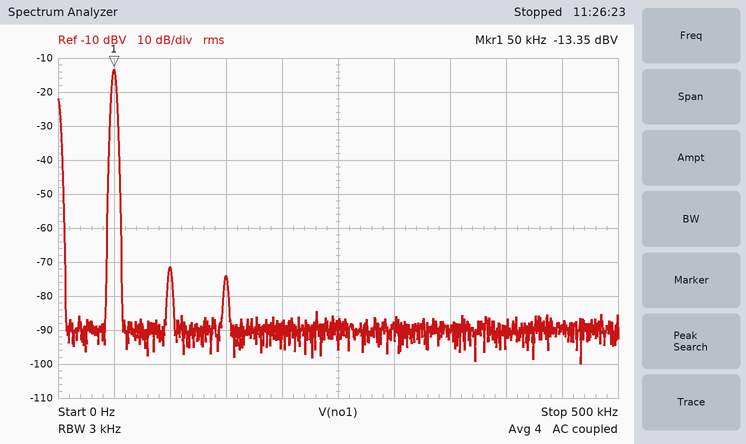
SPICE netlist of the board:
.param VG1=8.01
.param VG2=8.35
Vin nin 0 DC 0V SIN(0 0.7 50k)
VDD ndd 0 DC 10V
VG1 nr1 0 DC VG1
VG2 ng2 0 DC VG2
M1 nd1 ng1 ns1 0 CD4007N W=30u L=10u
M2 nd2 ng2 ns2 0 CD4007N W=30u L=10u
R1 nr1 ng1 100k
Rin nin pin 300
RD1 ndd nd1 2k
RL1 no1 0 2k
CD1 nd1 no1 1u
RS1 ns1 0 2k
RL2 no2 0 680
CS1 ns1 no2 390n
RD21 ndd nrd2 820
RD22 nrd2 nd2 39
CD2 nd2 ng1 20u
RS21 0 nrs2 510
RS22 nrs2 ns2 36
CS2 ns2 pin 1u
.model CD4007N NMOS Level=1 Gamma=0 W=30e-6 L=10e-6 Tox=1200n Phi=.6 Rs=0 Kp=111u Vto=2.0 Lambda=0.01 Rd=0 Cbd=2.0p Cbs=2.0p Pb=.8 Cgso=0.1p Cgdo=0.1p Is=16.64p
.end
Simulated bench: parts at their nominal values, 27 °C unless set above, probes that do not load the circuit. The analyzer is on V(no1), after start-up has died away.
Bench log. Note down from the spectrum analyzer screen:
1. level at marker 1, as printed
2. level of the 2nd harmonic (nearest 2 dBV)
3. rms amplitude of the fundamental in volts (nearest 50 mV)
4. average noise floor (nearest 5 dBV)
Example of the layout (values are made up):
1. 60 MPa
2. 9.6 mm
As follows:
1. -13.35 dBV
2. -72 dBV
3. 200 mV
4. -90 dBV
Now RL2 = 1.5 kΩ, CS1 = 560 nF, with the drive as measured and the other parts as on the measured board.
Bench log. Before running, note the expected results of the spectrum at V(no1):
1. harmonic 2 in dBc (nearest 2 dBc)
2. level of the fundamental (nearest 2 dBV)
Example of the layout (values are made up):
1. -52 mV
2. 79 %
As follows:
1. -48 dBc
2. -16 dBV
